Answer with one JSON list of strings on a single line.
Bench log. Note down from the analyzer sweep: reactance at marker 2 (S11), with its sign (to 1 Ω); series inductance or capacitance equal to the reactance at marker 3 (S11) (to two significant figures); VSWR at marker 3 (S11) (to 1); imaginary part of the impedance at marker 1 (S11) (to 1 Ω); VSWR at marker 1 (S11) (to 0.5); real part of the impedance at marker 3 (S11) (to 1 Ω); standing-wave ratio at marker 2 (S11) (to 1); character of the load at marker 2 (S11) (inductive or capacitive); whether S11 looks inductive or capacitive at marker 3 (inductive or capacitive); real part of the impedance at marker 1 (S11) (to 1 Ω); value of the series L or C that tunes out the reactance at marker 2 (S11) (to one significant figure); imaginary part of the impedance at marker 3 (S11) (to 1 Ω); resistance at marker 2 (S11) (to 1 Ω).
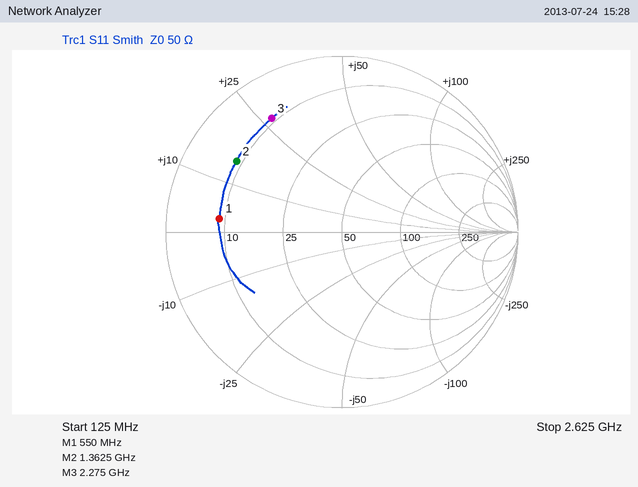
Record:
["+15 Ω", "1.9 nH", "7", "+3 Ω", "5.5", "9 Ω", "6", "inductive", "inductive", "9 Ω", "8 pF", "+27 Ω", "9 Ω"]
